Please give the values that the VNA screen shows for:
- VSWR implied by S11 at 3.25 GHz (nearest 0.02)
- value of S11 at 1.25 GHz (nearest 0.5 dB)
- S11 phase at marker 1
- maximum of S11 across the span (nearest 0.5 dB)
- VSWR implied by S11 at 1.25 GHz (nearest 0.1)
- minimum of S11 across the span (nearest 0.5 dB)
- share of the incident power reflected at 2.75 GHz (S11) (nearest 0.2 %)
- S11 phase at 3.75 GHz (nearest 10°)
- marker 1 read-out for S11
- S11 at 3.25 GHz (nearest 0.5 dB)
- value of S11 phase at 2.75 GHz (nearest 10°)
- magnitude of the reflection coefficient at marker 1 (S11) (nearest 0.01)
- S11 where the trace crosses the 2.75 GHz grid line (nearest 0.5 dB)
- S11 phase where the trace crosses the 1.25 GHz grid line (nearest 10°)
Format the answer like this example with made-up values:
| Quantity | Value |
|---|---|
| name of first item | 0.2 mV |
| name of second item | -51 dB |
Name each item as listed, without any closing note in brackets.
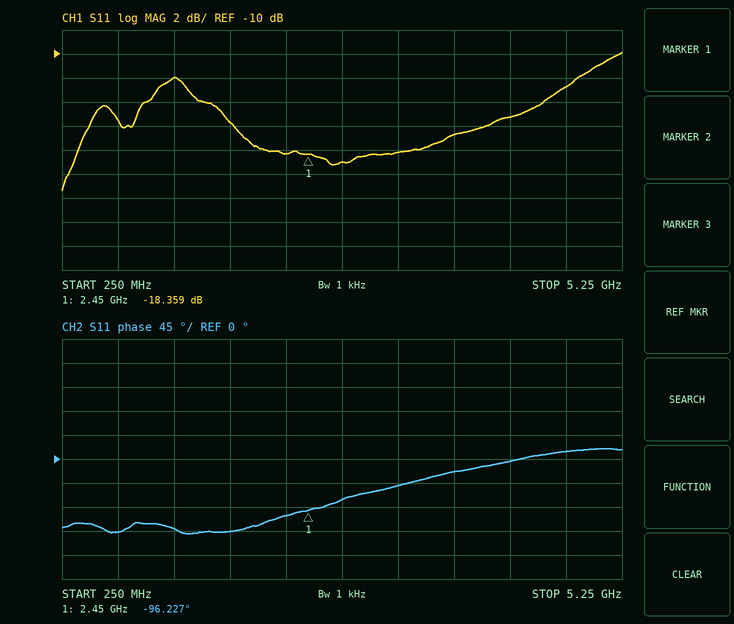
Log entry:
| Quantity | Value |
|---|---|
| VSWR implied by S11 at 3.25 GHz | 1.28 |
| value of S11 at 1.25 GHz | -12.0 dB |
| S11 phase at marker 1 | -96.227° |
| maximum of S11 across the span | -10.0 dB |
| VSWR implied by S11 at 1.25 GHz | 1.7 |
| minimum of S11 across the span | -21.5 dB |
| share of the incident power reflected at 2.75 GHz (S11) | 1.2 % |
| S11 phase at 3.75 GHz | -20° |
| marker 1 read-out for S11 | -18.359 dB |
| S11 at 3.25 GHz | -18.0 dB |
| value of S11 phase at 2.75 GHz | -80° |
| magnitude of the reflection coefficient at marker 1 (S11) | 0.12 |
| S11 where the trace crosses the 2.75 GHz grid line | -19.0 dB |
| S11 phase where the trace crosses the 1.25 GHz grid line | -130° |
